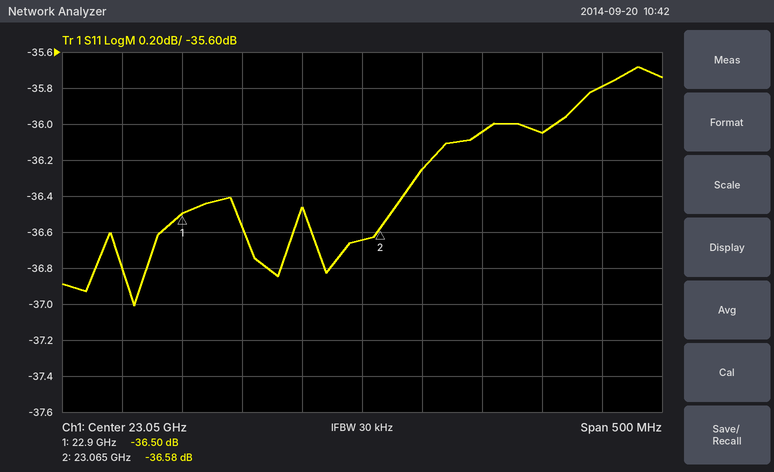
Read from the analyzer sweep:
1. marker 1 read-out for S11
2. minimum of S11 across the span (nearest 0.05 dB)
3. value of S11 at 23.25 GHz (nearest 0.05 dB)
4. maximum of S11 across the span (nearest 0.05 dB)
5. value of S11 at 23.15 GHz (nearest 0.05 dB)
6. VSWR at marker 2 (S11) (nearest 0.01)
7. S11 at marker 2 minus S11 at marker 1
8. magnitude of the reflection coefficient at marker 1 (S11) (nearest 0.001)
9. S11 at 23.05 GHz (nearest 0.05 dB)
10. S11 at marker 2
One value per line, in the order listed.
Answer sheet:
-36.50 dB
-37.00 dB
-35.80 dB
-35.70 dB
-36.05 dB
1.03
-0.08 dB
0.015
-36.65 dB
-36.58 dB
